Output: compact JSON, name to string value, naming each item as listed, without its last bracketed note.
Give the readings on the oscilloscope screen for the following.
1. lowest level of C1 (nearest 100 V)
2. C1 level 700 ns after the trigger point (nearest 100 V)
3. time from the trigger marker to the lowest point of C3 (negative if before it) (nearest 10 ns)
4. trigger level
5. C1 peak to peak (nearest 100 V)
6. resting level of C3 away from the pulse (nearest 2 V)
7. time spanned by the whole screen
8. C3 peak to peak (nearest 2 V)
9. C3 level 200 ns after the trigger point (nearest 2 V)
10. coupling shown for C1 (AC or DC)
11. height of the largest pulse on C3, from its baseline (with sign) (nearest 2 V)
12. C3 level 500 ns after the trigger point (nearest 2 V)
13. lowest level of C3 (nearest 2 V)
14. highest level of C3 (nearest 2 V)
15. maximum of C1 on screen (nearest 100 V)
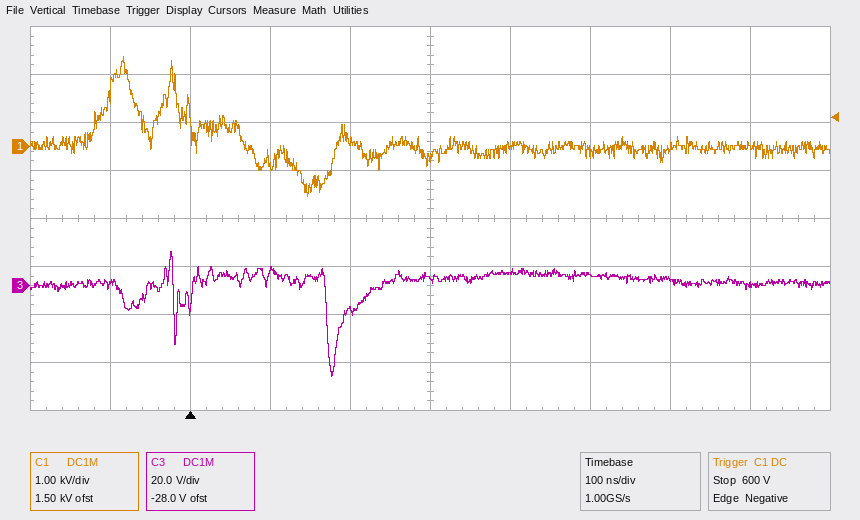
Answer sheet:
{"lowest level of C1": "-1.0 kV", "C1 level 700 ns after the trigger point": "0.0 kV", "time from the trigger marker to the lowest point of C3 (negative if before it)": "+180 ns", "trigger level": "600 V", "C1 peak to peak": "2.9 kV", "resting level of C3 away from the pulse": "2 V", "time spanned by the whole screen": "1 µs", "C3 peak to peak": "52 V", "C3 level 200 ns after the trigger point": "-10 V", "coupling shown for C1": "DC", "height of the largest pulse on C3, from its baseline (with sign)": "-40 V", "C3 level 500 ns after the trigger point": "4 V", "lowest level of C3": "-38 V", "highest level of C3": "14 V", "maximum of C1 on screen": "1.9 kV"}
